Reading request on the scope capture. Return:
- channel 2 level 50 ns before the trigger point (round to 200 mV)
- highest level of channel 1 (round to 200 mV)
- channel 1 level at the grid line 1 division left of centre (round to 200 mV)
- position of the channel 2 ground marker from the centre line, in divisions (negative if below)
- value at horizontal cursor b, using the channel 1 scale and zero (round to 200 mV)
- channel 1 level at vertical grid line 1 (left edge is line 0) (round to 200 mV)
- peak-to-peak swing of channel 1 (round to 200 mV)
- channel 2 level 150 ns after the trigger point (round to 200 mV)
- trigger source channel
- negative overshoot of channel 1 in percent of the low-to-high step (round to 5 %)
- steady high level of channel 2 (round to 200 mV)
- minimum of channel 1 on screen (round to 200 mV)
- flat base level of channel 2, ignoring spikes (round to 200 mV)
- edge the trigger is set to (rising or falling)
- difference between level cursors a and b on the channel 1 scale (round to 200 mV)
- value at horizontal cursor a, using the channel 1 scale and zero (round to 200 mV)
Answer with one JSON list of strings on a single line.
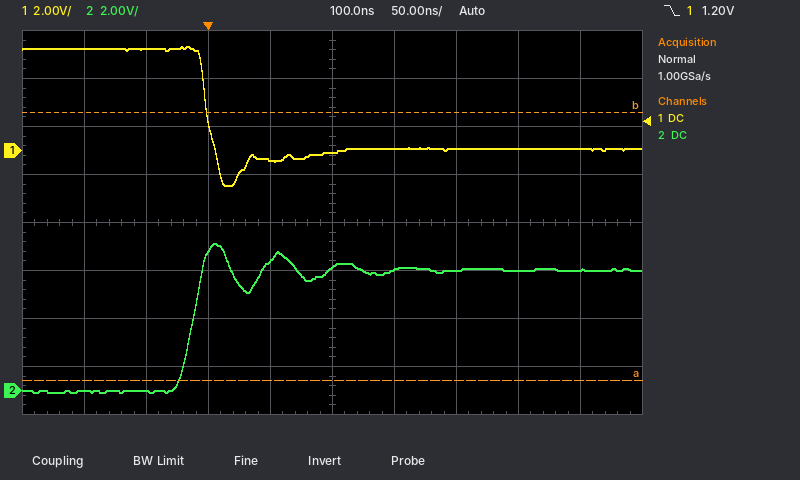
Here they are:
["0.0 V", "4.4 V", "-400 mV", "-3.5 div", "1.6 V", "4.2 V", "5.8 V", "5.0 V", "channel 1", "35 %", "5.0 V", "-1.4 V", "0.0 V", "falling", "11.2 V", "-9.6 V"]
